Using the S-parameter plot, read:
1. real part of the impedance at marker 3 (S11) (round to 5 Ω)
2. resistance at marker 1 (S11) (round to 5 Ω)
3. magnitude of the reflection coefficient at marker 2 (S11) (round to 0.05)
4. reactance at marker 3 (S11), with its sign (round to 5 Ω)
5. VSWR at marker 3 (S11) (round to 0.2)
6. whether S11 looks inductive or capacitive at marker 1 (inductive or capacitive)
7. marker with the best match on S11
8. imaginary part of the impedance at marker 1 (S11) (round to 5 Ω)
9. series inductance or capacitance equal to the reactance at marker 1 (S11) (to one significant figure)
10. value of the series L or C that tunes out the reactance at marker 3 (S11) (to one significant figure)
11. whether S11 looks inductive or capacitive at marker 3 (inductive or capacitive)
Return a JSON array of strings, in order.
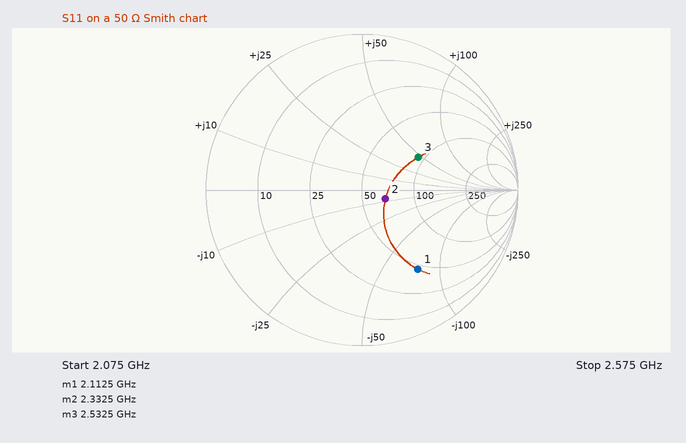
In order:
["90 Ω", "45 Ω", "0.15", "+45 Ω", "2.4", "capacitive", "marker 2", "-75 Ω", "1.0 pF", "1 pF", "inductive"]
